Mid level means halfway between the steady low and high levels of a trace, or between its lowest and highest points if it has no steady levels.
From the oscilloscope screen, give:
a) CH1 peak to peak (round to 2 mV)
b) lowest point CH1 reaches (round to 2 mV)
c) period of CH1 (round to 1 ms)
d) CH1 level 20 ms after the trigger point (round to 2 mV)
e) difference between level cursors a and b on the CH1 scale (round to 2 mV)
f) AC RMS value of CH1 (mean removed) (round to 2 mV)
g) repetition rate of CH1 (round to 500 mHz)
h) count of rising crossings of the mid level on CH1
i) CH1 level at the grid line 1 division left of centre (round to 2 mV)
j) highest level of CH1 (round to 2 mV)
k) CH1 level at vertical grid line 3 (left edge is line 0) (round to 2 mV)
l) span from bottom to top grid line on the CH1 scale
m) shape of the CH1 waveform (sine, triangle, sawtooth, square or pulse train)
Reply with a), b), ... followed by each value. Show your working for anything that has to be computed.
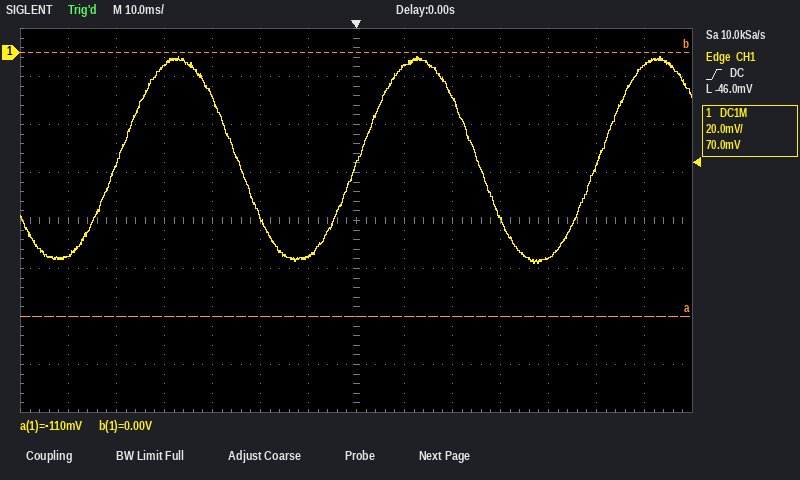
a) -2 mV − (-88 mV) = 86 mV
b) -88 mV
c) 50 ms
d) -18 mV
e) 110 mV
f) 86 mV / (2√2) ≈ 30 mV
g) 1 / 50 ms ≈ 20.0 Hz
h) 3
i) -84 mV
j) -2 mV
k) -6 mV
l) 160 mV
m) sine
